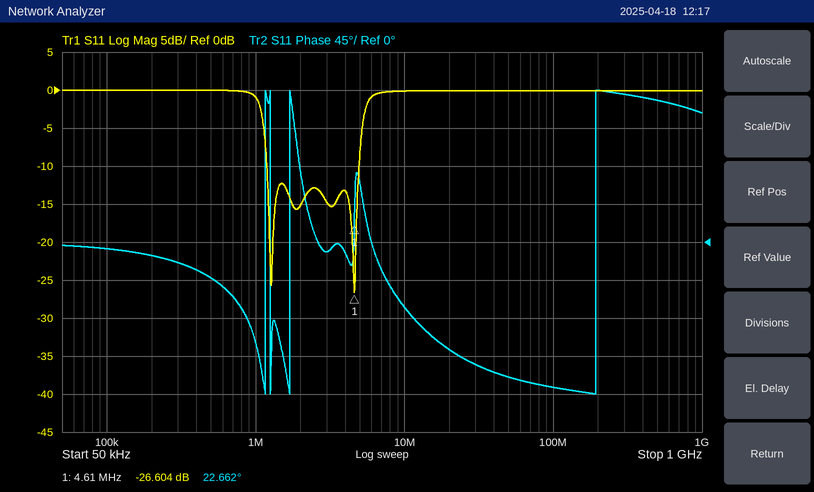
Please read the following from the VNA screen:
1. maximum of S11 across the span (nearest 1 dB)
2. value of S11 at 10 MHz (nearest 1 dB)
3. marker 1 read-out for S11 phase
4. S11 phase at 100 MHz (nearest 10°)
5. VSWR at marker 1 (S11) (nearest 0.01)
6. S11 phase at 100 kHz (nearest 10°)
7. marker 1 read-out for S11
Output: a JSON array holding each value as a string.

["0 dB", "0 dB", "22.662°", "-170°", "1.10", "-10°", "-26.604 dB"]
